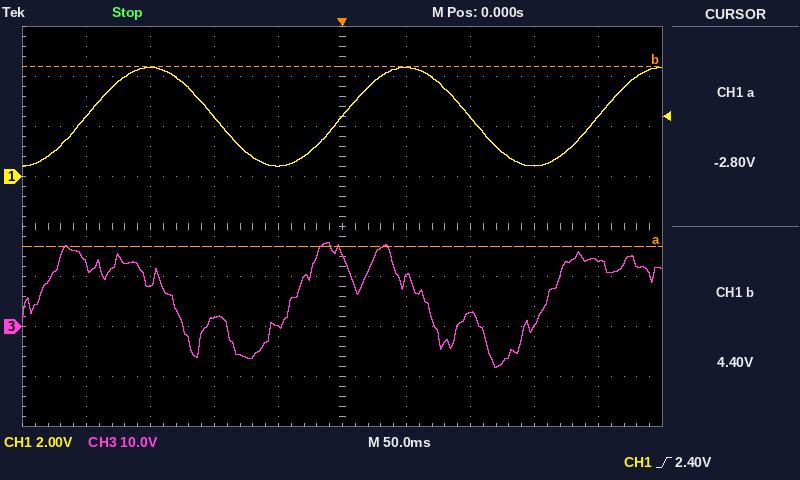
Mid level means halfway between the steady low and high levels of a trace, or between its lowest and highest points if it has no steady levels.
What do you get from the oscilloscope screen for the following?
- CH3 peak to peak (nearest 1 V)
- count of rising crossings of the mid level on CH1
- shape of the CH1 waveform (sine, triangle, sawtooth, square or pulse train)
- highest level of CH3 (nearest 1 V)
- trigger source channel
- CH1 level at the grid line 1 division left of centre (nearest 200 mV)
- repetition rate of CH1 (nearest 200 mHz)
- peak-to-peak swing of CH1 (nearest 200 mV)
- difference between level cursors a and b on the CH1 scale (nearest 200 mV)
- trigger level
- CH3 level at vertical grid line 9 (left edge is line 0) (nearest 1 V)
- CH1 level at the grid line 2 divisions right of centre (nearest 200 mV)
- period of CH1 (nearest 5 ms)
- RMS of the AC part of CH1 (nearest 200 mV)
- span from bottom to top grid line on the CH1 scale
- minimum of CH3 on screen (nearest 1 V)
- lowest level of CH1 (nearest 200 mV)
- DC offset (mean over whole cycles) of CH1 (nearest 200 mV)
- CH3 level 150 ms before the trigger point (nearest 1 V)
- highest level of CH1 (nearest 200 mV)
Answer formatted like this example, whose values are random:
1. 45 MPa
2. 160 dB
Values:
1. 25 V
2. 3
3. sine
4. 17 V
5. CH1
6. 400 mV
7. 5.0 Hz
8. 4.0 V
9. 7.2 V
10. 2.40 V
11. 13 V
12. 2.4 V
13. 200 ms
14. 1.4 V
15. 16 V
16. -8 V
17. 400 mV
18. 2.4 V
19. 8 V
20. 4.4 V
